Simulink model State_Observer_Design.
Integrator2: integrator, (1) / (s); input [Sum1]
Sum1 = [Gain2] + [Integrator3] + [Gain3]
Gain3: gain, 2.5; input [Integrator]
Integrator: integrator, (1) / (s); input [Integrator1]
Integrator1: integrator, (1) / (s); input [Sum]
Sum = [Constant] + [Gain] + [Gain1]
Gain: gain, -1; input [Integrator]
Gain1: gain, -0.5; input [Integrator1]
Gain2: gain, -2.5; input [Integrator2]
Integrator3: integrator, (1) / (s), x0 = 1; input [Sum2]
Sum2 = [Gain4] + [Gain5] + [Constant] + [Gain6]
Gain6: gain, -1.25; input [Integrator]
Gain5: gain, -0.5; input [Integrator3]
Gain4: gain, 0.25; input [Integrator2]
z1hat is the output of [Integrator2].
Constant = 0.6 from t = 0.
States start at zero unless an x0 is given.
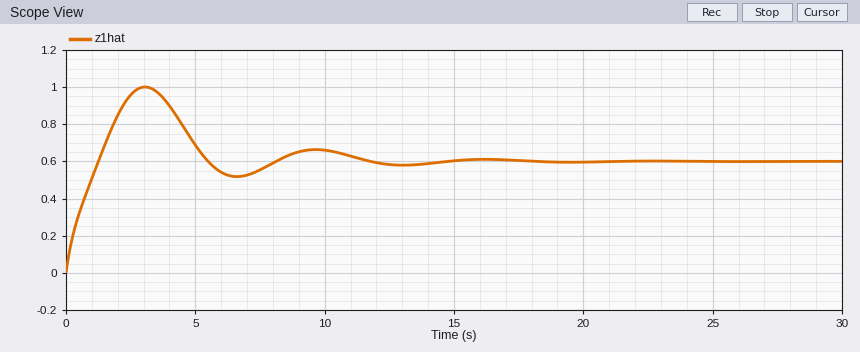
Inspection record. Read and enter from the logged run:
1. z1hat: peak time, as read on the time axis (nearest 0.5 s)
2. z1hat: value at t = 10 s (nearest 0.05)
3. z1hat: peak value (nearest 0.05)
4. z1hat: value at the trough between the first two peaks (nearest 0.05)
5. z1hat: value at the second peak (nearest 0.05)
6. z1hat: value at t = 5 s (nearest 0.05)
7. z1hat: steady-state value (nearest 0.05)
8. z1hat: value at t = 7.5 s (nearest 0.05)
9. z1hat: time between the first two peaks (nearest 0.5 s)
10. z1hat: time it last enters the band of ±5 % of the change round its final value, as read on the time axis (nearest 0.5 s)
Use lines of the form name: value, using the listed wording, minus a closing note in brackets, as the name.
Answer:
z1hat: peak time, as read on the time axis: 3.0 s
z1hat: value at t = 10 s: 0.65
z1hat: peak value: 1.00
z1hat: value at the trough between the first two peaks: 0.50
z1hat: value at the second peak: 0.65
z1hat: value at t = 5 s: 0.70
z1hat: steady-state value: 0.60
z1hat: value at t = 7.5 s: 0.55
z1hat: time between the first two peaks: 6.5 s
z1hat: time it last enters the band of ±5 % of the change round its final value, as read on the time axis: 11.0 s
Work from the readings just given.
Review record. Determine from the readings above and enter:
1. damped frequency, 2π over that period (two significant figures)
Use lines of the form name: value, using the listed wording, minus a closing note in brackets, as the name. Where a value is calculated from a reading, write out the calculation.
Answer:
damped frequency, 2π over that period: 2π / 6.5 = 0.97 rad/s
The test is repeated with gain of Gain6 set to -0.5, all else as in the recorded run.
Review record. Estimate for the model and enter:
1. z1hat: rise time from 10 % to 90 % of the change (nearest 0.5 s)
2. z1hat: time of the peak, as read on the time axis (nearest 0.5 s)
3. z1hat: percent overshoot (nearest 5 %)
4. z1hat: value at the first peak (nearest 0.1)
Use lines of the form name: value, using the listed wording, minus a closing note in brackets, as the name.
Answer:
z1hat: rise time from 10 % to 90 % of the change: 2.0 s
z1hat: time of the peak, as read on the time axis: 3.5 s
z1hat: percent overshoot: 20 %
z1hat: value at the first peak: 1.3
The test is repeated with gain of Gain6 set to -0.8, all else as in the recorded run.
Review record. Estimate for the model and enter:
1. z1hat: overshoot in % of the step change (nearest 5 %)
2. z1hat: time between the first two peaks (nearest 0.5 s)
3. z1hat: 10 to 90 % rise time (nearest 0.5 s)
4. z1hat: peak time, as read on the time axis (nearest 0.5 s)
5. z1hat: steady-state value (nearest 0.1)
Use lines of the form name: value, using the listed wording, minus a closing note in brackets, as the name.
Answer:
z1hat: overshoot in % of the step change: 30 %
z1hat: time between the first two peaks: 6.5 s
z1hat: 10 to 90 % rise time: 1.5 s
z1hat: peak time, as read on the time axis: 3.5 s
z1hat: steady-state value: 0.9
